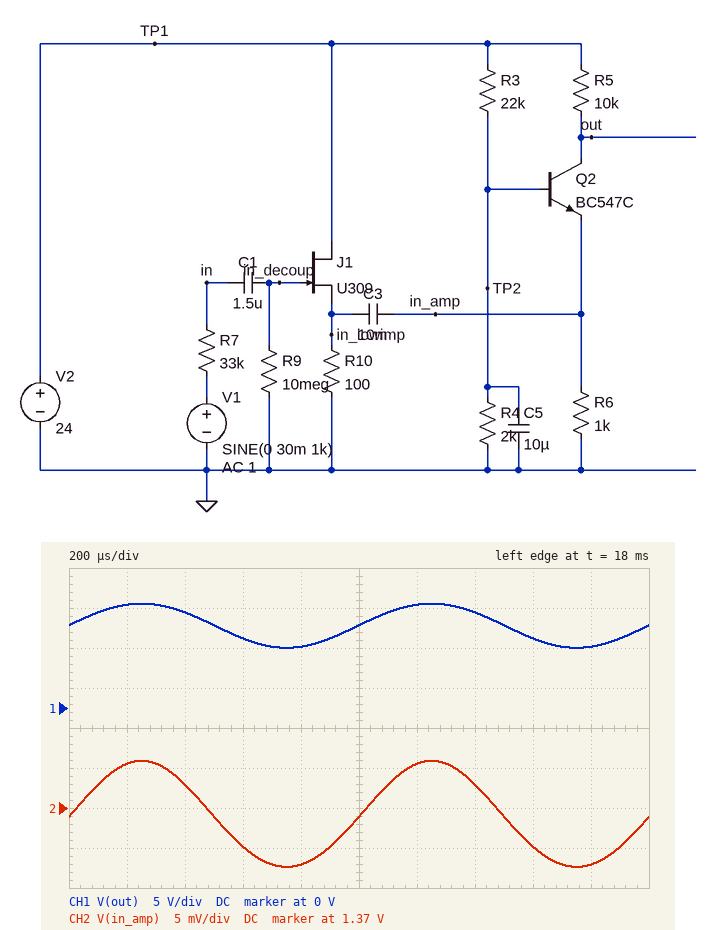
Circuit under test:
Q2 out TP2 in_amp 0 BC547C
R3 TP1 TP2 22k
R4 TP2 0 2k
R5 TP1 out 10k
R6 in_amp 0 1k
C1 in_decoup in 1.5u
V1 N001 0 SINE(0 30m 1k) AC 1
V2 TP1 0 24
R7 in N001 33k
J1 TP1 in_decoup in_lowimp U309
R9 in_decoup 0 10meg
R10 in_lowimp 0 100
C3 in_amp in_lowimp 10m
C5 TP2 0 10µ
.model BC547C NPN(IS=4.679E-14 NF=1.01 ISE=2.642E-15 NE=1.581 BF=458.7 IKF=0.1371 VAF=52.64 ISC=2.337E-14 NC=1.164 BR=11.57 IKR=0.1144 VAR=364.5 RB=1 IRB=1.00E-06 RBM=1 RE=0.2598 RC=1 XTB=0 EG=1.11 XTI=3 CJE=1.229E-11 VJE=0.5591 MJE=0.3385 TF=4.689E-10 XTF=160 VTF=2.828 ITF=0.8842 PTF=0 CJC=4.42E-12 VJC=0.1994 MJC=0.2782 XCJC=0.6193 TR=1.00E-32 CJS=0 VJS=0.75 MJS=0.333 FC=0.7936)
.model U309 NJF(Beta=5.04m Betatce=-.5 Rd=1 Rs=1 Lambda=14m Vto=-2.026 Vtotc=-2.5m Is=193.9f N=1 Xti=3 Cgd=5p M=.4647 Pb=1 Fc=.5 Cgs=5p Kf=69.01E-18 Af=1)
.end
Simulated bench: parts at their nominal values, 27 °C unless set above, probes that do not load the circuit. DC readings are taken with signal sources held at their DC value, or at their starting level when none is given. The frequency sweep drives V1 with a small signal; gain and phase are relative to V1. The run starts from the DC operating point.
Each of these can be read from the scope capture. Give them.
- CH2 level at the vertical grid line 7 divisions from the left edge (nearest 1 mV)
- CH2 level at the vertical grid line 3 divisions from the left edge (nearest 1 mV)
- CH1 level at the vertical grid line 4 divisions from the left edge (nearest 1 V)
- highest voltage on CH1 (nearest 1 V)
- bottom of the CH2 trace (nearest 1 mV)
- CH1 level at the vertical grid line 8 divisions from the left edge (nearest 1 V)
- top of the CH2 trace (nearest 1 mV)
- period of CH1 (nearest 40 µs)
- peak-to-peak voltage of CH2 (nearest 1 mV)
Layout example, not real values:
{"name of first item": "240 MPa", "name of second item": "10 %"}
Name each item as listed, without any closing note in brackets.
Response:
{"CH2 level at the vertical grid line 7 divisions from the left edge": "1.373 V", "CH2 level at the vertical grid line 3 divisions from the left edge": "1.365 V", "CH1 level at the vertical grid line 4 divisions from the left edge": "8 V", "highest voltage on CH1": "13 V", "bottom of the CH2 trace": "1.363 V", "CH1 level at the vertical grid line 8 divisions from the left edge": "9 V", "top of the CH2 trace": "1.376 V", "period of CH1": "1.00 ms", "peak-to-peak voltage of CH2": "13 mV"}
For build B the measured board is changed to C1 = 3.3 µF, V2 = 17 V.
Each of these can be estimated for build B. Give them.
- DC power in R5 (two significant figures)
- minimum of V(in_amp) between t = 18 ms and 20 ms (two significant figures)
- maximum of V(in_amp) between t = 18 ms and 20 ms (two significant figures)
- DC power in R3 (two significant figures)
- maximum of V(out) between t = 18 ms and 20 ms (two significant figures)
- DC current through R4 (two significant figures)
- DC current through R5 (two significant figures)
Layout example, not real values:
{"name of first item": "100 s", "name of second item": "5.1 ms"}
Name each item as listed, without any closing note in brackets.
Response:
{"DC power in R5": "6.4 mW", "minimum of V(in_amp) between t = 18 ms and 20 ms": "790 mV", "maximum of V(in_amp) between t = 18 ms and 20 ms": "810 mV", "DC power in R3": "11 mW", "maximum of V(out) between t = 18 ms and 20 ms": "11 V", "DC current through R4": "710 µA", "DC current through R5": "800 µA"}
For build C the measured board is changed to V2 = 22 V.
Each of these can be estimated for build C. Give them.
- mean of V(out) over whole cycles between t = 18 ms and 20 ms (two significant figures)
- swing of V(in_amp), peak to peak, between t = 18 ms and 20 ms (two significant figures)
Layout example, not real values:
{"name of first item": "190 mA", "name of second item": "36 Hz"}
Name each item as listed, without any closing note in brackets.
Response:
{"mean of V(out) over whole cycles between t = 18 ms and 20 ms": "9.9 V", "swing of V(in_amp), peak to peak, between t = 18 ms and 20 ms": "14 mV"}
